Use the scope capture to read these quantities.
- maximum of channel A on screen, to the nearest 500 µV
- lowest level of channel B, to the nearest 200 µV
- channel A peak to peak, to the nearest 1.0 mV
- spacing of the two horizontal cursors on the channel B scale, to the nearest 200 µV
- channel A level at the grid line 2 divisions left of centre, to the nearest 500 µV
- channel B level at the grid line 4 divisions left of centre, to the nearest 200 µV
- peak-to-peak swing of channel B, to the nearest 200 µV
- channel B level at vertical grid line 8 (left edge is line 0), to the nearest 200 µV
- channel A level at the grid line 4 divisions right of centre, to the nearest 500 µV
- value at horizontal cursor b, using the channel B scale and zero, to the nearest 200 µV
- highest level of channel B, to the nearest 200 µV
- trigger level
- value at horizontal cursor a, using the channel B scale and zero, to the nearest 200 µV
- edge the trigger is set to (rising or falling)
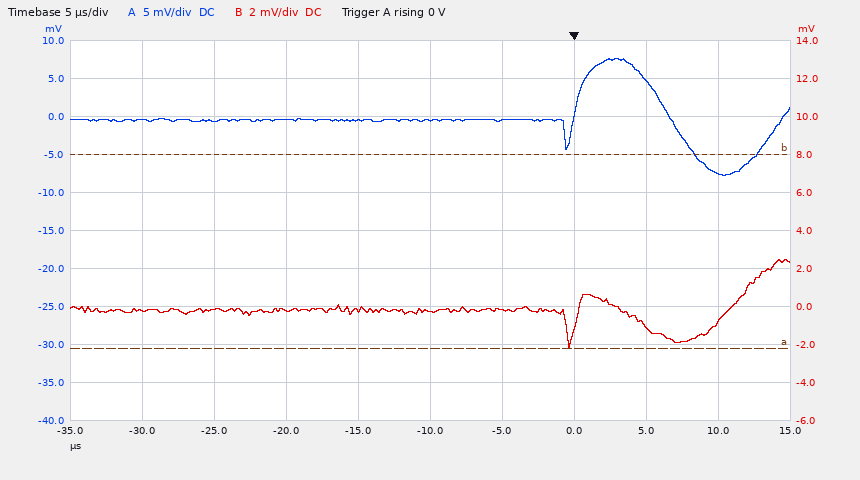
7.5 mV
-2.2 mV
15.0 mV
10.2 mV
-500 µV
-200 µV
4.6 mV
-1.0 mV
-7.5 mV
8.0 mV
2.4 mV
0 V
-2.2 mV
rising
